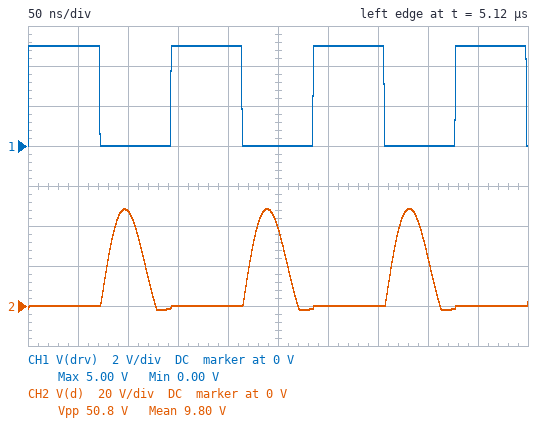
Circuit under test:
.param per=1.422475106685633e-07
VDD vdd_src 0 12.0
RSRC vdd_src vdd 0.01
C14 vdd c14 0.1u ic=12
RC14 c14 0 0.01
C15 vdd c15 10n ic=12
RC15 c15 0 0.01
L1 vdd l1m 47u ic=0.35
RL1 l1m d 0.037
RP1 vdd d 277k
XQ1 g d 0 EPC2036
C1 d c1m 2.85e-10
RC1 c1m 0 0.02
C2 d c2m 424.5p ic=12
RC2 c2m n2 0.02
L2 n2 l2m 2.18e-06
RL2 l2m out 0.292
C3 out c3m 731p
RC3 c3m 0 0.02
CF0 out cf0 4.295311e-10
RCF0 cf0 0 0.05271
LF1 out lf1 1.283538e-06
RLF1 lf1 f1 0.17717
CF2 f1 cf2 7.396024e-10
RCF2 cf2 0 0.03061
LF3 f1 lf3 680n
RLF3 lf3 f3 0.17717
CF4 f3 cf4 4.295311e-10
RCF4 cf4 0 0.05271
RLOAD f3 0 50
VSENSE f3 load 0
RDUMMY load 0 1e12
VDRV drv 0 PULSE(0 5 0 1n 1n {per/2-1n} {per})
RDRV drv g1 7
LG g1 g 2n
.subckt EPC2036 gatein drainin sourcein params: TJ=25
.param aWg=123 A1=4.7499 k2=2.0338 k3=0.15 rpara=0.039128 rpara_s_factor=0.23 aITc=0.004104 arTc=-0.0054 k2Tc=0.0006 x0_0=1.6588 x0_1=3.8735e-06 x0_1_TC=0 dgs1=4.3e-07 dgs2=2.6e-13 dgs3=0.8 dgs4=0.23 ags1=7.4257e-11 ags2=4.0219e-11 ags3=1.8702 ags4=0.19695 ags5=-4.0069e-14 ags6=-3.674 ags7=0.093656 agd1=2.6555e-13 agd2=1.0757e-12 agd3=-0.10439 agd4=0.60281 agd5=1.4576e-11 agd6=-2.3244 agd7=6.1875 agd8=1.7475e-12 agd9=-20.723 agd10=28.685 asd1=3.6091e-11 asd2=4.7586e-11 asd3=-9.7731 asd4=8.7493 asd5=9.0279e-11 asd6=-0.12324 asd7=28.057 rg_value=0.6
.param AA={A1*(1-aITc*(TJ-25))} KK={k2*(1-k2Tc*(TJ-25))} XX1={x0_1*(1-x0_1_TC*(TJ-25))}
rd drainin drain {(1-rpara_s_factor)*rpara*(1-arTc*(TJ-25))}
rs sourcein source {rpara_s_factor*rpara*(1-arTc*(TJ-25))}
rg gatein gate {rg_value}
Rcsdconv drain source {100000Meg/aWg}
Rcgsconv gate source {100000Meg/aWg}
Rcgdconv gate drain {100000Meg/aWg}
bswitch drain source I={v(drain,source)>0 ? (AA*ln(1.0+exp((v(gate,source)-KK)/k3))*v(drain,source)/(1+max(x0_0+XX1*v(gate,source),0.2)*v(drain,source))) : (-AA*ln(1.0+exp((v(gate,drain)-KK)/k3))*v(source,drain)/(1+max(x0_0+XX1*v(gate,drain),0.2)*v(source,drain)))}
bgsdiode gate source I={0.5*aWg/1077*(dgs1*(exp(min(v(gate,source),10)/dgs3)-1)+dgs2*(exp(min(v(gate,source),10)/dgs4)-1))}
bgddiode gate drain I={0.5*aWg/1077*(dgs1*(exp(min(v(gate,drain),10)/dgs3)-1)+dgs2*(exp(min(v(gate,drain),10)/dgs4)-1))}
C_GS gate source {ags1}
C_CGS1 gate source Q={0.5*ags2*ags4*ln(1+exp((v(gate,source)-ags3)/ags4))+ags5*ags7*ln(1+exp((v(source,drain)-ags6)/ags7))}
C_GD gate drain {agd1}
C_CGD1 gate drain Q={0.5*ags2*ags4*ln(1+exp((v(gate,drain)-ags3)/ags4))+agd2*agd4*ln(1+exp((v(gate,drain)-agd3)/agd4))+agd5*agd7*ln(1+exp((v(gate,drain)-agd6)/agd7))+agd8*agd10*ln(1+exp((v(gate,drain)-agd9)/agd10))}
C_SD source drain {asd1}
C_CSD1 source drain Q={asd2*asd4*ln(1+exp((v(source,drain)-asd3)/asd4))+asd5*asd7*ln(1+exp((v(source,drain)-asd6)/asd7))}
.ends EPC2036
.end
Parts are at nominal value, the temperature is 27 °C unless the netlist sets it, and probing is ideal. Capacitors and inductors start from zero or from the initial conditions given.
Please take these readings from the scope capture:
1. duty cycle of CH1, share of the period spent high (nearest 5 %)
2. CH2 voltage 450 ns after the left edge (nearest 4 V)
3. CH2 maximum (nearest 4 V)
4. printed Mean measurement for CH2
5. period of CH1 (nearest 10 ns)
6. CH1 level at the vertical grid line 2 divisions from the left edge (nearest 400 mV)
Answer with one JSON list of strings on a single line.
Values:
["50 %", "0 V", "48 V", "9.80 V", "140 ns", "0 V"]
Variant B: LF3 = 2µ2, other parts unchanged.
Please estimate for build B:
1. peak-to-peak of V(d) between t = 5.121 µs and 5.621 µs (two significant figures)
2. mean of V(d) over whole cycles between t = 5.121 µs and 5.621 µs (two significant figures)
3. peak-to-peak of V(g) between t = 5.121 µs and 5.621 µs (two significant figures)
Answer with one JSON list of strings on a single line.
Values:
["34 V", "12 V", "5.0 V"]
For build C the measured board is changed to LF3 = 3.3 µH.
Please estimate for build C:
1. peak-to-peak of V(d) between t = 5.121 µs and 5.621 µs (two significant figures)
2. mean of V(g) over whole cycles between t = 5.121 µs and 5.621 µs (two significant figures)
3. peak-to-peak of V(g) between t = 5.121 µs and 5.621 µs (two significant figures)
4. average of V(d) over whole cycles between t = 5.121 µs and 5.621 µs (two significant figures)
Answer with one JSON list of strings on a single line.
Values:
["35 V", "2.5 V", "5.0 V", "12 V"]
